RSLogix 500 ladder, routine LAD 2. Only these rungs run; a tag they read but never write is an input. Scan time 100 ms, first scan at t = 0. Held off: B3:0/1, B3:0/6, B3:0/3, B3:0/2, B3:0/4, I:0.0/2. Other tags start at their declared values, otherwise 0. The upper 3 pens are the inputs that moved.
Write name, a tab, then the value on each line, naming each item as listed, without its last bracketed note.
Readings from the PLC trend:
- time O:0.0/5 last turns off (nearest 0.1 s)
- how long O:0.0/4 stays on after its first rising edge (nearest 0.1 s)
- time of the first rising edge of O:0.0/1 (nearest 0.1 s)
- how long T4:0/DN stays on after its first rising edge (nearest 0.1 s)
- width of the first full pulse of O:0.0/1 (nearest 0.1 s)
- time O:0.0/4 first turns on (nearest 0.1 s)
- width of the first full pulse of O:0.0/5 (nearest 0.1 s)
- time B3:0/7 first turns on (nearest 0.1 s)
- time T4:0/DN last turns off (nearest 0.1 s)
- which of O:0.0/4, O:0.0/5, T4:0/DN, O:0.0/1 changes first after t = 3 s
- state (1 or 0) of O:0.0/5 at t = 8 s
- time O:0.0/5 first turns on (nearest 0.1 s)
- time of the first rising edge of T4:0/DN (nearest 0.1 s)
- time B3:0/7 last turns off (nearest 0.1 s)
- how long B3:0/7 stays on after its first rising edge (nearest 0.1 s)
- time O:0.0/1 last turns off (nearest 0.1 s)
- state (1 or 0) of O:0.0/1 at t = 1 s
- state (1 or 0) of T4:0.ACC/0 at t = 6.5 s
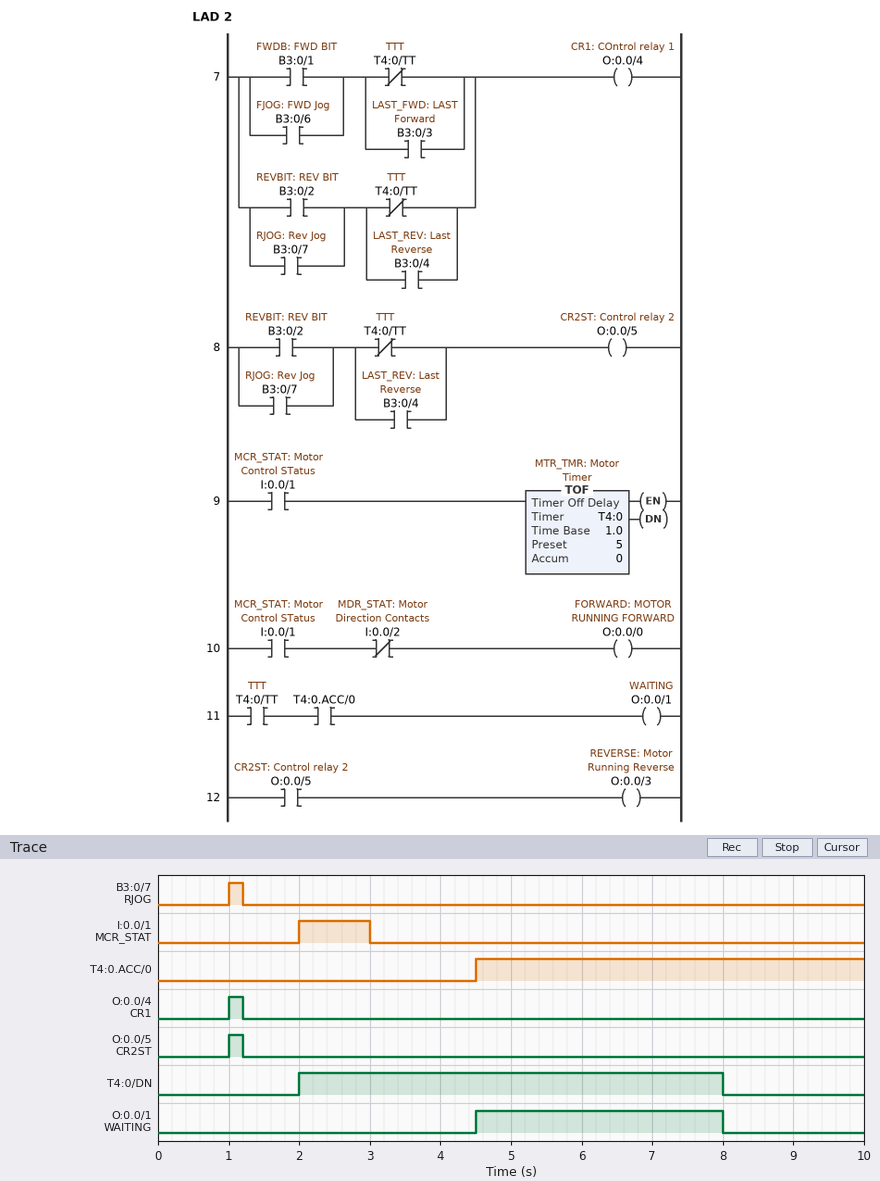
time O:0.0/5 last turns off	1.2 s
how long O:0.0/4 stays on after its first rising edge	0.2 s
time of the first rising edge of O:0.0/1	4.5 s
how long T4:0/DN stays on after its first rising edge	6.0 s
width of the first full pulse of O:0.0/1	3.5 s
time O:0.0/4 first turns on	1.0 s
width of the first full pulse of O:0.0/5	0.2 s
time B3:0/7 first turns on	1.0 s
time T4:0/DN last turns off	8.0 s
which of O:0.0/4, O:0.0/5, T4:0/DN, O:0.0/1 changes first after t = 3 s	O:0.0/1
state (1 or 0) of O:0.0/5 at t = 8 s	0
time O:0.0/5 first turns on	1.0 s
time of the first rising edge of T4:0/DN	2.0 s
time B3:0/7 last turns off	1.2 s
how long B3:0/7 stays on after its first rising edge	0.2 s
time O:0.0/1 last turns off	8.0 s
state (1 or 0) of O:0.0/1 at t = 1 s	0
state (1 or 0) of T4:0.ACC/0 at t = 6.5 s	1
